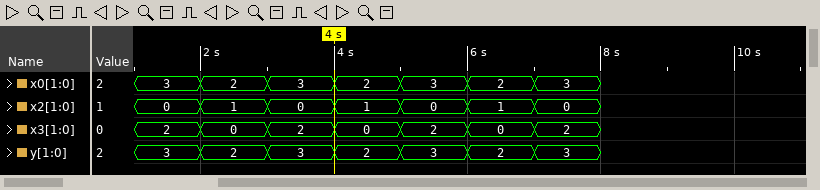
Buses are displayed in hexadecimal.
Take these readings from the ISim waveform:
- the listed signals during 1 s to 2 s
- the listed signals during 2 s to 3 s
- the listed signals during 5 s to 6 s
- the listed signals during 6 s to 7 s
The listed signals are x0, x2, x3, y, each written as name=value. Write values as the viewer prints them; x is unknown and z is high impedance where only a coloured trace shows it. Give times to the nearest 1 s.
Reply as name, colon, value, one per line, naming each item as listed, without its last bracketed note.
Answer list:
the listed signals during 1 s to 2 s: x0=3, x2=0, x3=2, y=3
the listed signals during 2 s to 3 s: x0=2, x2=1, x3=0, y=2
the listed signals during 5 s to 6 s: x0=3, x2=0, x3=2, y=3
the listed signals during 6 s to 7 s: x0=2, x2=1, x3=0, y=2
